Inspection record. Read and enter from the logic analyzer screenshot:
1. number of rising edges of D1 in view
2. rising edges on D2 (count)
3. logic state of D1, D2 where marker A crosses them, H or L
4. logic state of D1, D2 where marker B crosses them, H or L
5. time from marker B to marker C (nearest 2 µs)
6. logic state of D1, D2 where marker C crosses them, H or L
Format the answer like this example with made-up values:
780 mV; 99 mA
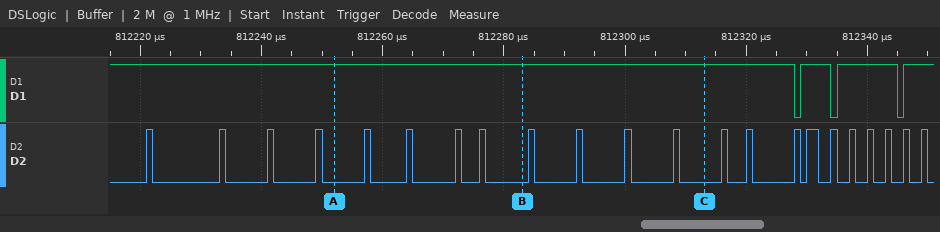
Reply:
3; 22; D1=H, D2=L; D1=H, D2=L; 30 µs; D1=H, D2=L
